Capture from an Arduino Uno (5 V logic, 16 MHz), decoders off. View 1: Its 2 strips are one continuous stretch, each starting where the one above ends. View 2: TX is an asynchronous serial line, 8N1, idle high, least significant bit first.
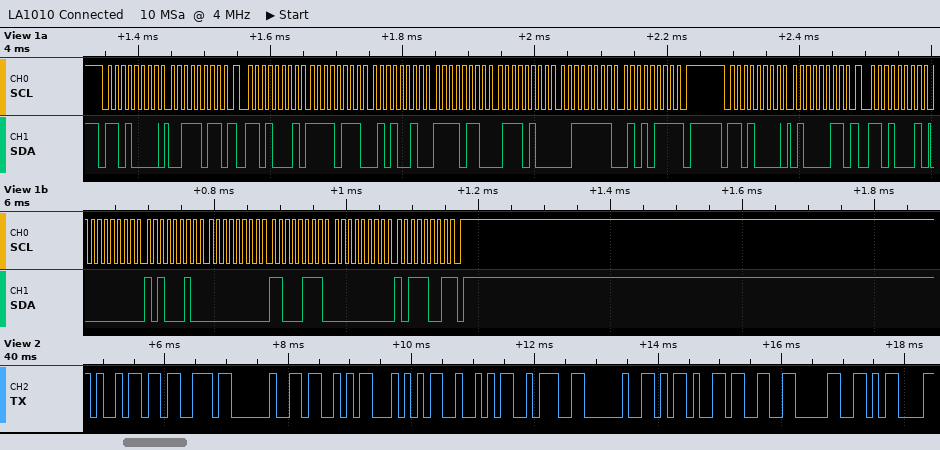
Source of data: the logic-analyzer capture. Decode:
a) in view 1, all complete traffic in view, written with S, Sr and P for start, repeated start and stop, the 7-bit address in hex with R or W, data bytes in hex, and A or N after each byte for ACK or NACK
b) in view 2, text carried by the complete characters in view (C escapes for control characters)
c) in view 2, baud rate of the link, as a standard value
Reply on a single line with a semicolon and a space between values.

S 68W A 3B A Sr 68R A F7 A 52 A F6 A 74 A 3F A 57 N P S 68W A 43 A Sr 68R A 00 A A2 A 00 A C7 A 00 A B9 N P; "is STR: -30\r"; 9600 baud
